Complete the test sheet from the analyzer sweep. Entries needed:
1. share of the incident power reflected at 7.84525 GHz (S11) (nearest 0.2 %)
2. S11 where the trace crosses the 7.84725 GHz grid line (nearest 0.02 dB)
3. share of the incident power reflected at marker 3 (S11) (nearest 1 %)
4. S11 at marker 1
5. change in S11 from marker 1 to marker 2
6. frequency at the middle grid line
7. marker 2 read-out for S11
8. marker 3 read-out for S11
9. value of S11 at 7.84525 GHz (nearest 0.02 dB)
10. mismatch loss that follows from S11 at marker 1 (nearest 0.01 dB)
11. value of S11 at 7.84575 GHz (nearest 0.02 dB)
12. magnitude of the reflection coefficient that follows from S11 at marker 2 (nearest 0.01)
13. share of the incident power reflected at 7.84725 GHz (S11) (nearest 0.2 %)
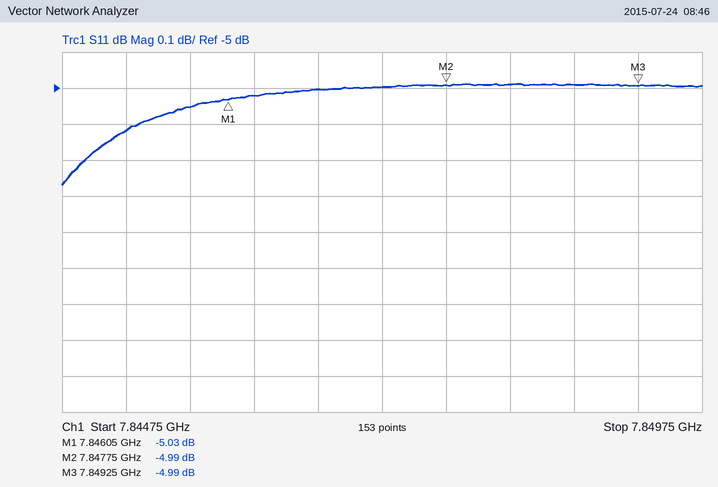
30.8 %
-5.00 dB
32 %
-5.03 dB
0.04 dB
7.84725 GHz
-4.99 dB
-4.99 dB
-5.12 dB
1.64 dB
-5.06 dB
0.56
31.6 %
